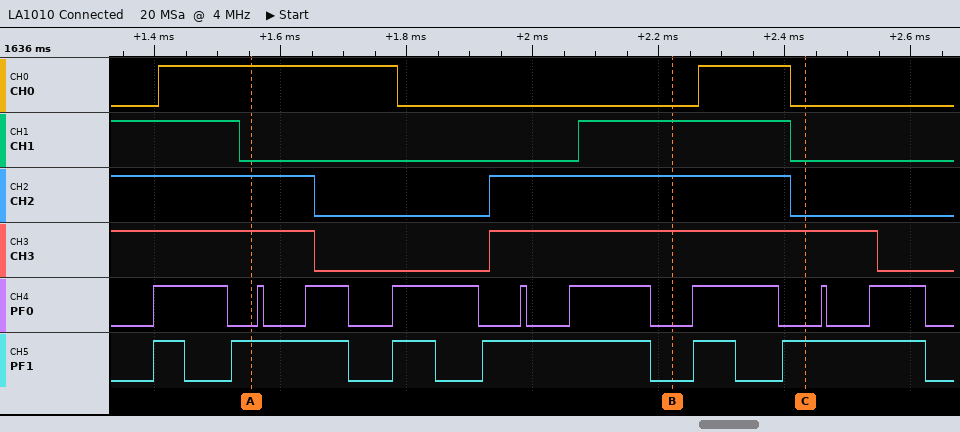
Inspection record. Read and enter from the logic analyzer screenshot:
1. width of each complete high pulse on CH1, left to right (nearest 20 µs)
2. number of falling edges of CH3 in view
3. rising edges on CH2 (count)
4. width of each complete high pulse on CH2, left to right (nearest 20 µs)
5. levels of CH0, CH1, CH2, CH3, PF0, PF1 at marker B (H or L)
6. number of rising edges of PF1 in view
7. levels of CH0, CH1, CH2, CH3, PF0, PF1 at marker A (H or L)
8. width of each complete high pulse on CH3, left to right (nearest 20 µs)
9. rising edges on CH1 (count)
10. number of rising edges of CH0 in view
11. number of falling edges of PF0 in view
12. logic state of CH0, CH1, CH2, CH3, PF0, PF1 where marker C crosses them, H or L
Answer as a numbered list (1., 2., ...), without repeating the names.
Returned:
1. 340 µs
2. 2
3. 1
4. 480 µs
5. CH0=L, CH1=H, CH2=H, CH3=H, PF0=L, PF1=L
6. 6
7. CH0=H, CH1=L, CH2=H, CH3=H, PF0=L, PF1=H
8. 620 µs
9. 1
10. 2
11. 9
12. CH0=L, CH1=L, CH2=L, CH3=H, PF0=L, PF1=H
